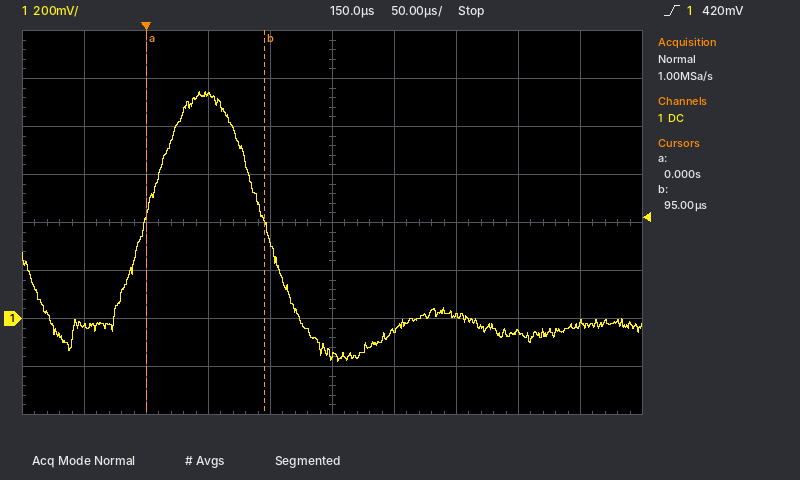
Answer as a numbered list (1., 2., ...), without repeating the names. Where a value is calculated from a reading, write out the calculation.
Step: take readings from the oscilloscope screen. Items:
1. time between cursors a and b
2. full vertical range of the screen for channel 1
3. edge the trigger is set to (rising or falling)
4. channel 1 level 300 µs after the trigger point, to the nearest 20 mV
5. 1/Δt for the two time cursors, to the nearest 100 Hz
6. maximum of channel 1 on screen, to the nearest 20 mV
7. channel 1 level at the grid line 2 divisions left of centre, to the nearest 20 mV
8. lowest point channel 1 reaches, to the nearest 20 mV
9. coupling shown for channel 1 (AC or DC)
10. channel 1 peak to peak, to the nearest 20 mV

1. 95 µs − (0 s) = 95 µs
2. 1.6 V
3. rising
4. -60 mV
5. 1 / 95 µs ≈ 10.5 kHz
6. 940 mV
7. 940 mV
8. -180 mV
9. DC
10. 940 mV − (-180 mV) = 1.12 V
